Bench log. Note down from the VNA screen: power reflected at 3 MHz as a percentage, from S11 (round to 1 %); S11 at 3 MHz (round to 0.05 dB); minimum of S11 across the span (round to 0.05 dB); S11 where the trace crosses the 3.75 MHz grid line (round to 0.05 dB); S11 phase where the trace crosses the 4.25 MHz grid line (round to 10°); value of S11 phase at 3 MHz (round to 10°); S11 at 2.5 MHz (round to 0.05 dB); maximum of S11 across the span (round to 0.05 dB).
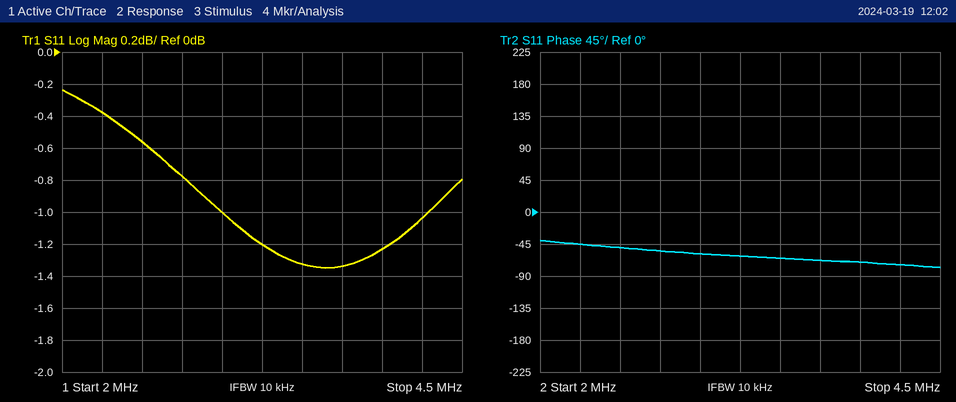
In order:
79 %
-1.00 dB
-1.35 dB
-1.35 dB
-70°
-60°
-0.55 dB
-0.25 dB
